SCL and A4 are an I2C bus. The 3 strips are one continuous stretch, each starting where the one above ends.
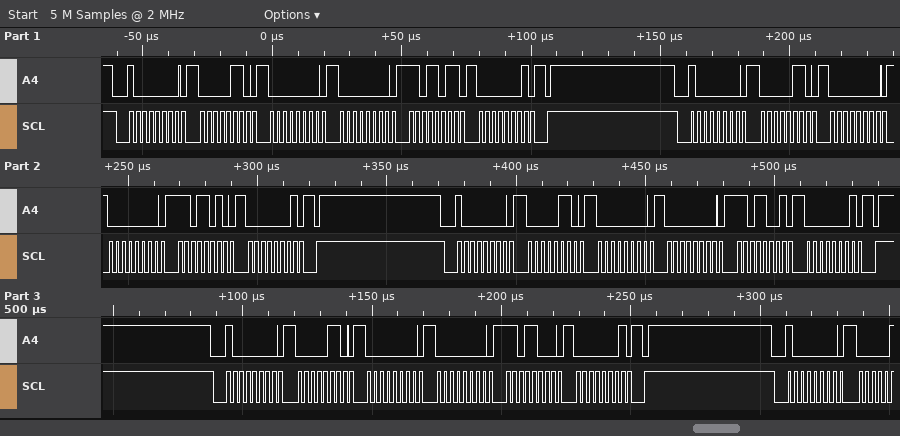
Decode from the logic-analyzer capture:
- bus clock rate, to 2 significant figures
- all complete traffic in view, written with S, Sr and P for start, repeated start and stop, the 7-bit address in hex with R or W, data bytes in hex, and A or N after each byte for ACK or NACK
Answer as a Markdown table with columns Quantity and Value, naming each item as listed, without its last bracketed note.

| Quantity | Value |
|---|---|
| bus clock rate, to 2 significant figures | 400 kHz |
| all complete traffic in view, written with S, Sr and P for start, repeated start and stop, the 7-bit address in hex with R or W, data bytes in hex, and A or N after each byte for ACK or NACK | S 40W A 06 A 00 A 00 A DB A 01 A P S 40W A 06 A 00 A 00 A DA A 01 A P S 40W A 06 A 00 A 00 A D9 A 01 A P S 40W A 06 A 00 A 00 A D8 A 01 A P S 40W A |
